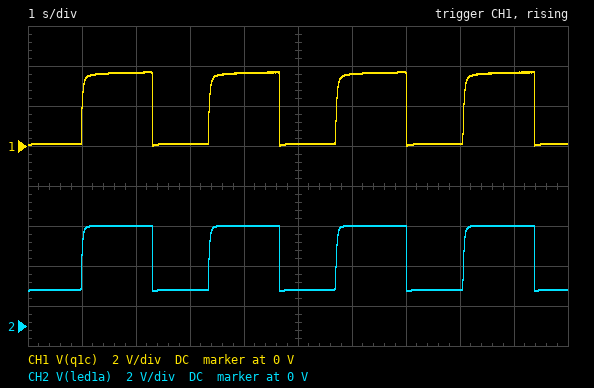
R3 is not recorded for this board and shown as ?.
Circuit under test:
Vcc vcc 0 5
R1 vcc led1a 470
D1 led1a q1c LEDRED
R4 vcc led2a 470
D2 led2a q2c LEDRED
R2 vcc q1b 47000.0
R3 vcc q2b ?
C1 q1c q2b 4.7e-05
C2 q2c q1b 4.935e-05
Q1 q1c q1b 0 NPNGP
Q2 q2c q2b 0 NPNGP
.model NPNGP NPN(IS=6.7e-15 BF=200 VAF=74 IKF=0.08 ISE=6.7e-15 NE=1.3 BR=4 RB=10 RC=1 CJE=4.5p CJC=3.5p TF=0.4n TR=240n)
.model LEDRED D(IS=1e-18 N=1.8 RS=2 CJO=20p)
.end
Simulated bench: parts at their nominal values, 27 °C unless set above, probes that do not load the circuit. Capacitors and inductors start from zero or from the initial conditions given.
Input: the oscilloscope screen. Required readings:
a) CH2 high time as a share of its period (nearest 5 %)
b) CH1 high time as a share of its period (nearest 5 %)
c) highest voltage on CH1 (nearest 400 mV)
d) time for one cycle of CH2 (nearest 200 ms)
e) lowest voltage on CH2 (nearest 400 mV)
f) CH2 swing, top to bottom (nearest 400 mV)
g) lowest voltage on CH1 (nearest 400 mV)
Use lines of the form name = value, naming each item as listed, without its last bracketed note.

CH2 high time as a share of its period = 55 %
CH1 high time as a share of its period = 55 %
highest voltage on CH1 = 3.6 V
time for one cycle of CH2 = 2.4 s
lowest voltage on CH2 = 1.6 V
CH2 swing, top to bottom = 3.2 V
lowest voltage on CH1 = 0 V
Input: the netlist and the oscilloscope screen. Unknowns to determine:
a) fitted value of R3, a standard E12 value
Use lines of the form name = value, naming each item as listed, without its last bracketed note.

fitted value of R3, a standard E12 value = 39 kΩ
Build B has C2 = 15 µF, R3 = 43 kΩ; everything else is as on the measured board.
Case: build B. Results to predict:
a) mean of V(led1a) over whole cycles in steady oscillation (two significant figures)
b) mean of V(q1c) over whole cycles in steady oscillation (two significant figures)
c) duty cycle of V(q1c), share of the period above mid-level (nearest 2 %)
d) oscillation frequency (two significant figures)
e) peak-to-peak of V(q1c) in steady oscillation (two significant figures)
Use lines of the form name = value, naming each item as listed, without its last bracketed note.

mean of V(led1a) over whole cycles in steady oscillation = 2.6 V
mean of V(q1c) over whole cycles in steady oscillation = 960 mV
duty cycle of V(q1c), share of the period above mid-level = 26 %
oscillation frequency = 650 mHz
peak-to-peak of V(q1c) in steady oscillation = 3.6 V
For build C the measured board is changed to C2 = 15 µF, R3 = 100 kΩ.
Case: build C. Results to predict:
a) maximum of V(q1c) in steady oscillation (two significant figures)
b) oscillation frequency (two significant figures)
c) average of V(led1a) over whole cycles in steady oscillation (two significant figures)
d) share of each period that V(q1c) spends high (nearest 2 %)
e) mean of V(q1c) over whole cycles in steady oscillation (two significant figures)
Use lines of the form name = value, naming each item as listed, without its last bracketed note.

maximum of V(q1c) in steady oscillation = 3.6 V
oscillation frequency = 330 mHz
average of V(led1a) over whole cycles in steady oscillation = 2.2 V
share of each period that V(q1c) spends high = 12 %
mean of V(q1c) over whole cycles in steady oscillation = 520 mV
